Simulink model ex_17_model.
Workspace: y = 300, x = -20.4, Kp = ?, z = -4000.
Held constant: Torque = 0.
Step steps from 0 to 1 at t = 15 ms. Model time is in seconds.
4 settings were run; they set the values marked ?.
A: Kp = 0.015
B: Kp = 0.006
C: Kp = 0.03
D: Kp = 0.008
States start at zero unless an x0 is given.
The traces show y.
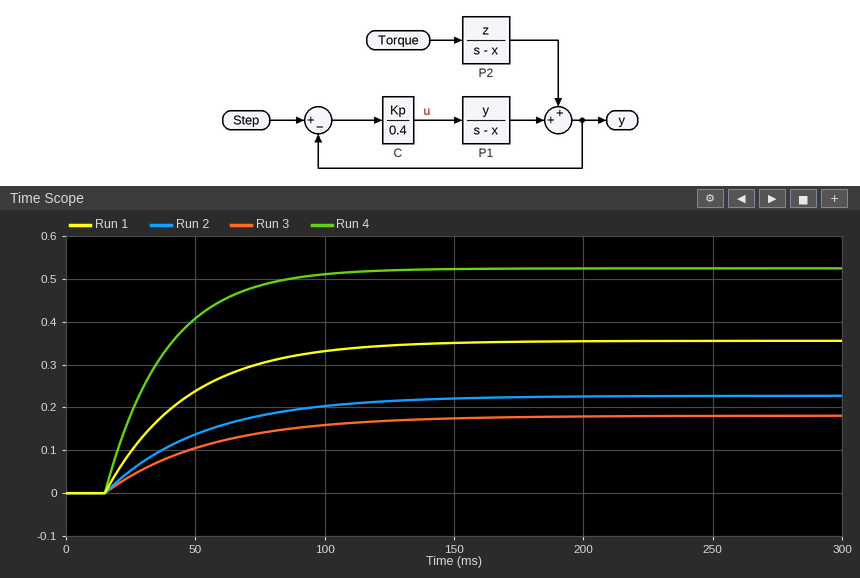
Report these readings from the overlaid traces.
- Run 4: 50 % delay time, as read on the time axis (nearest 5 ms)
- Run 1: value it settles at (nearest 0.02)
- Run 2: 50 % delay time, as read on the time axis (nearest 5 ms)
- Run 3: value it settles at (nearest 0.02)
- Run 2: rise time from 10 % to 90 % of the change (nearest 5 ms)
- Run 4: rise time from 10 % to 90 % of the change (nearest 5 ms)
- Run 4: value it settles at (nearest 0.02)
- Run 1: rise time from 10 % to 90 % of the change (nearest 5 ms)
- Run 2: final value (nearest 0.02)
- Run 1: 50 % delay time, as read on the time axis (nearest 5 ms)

30 ms
0.36
40 ms
0.18
85 ms
50 ms
0.52
70 ms
0.22
35 ms
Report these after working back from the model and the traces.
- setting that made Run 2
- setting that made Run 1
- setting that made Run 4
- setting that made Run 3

D
A
C
B
